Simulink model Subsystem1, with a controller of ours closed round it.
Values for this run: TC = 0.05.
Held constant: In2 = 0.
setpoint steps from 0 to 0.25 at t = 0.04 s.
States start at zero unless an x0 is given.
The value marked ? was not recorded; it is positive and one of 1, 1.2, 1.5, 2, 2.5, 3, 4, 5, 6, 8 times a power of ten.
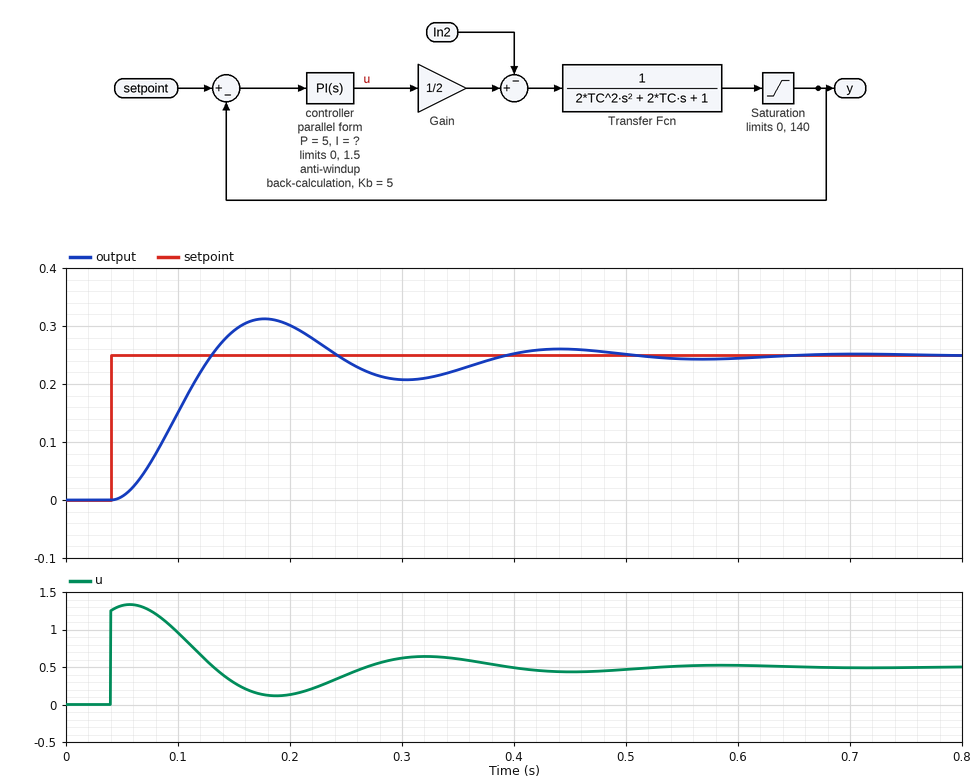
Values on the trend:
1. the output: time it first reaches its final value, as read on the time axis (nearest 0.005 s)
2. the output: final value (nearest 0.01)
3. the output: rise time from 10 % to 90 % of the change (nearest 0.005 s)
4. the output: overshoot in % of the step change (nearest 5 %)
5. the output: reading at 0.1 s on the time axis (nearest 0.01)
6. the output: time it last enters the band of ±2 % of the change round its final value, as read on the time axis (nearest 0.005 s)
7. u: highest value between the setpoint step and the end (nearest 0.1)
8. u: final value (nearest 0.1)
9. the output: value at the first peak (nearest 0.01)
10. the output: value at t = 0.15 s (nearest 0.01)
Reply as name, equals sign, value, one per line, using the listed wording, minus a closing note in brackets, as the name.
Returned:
the output: time it first reaches its final value, as read on the time axis = 0.130 s
the output: final value = 0.25
the output: rise time from 10 % to 90 % of the change = 0.060 s
the output: overshoot in % of the step change = 25 %
the output: reading at 0.1 s on the time axis = 0.15
the output: time it last enters the band of ±2 % of the change round its final value, as read on the time axis = 0.610 s
u: highest value between the setpoint step and the end = 1.3
u: final value = 0.5
the output: value at the first peak = 0.31
the output: value at t = 0.15 s = 0.29
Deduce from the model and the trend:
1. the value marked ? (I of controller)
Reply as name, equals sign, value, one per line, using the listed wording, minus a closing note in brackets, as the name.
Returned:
the value marked ? = 40
